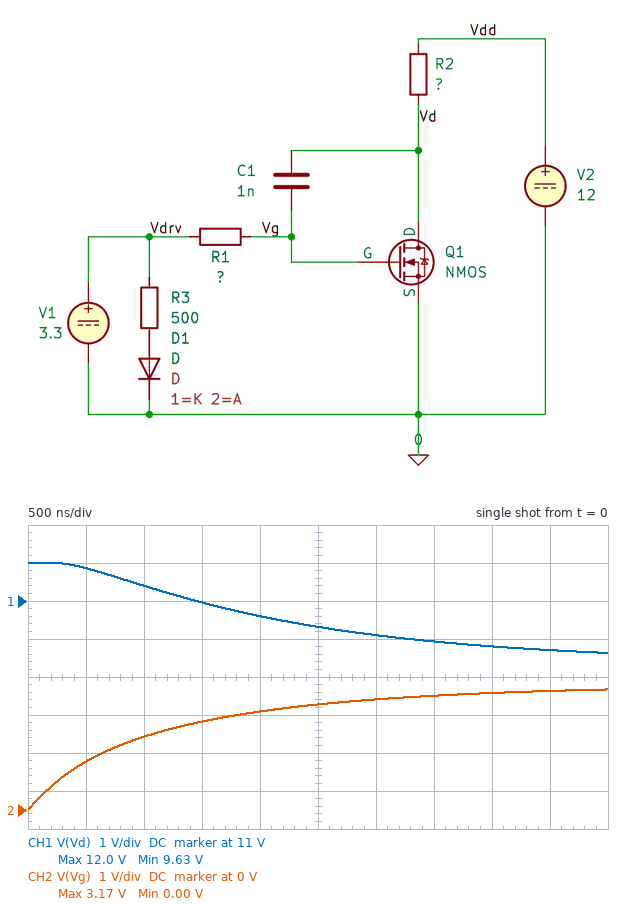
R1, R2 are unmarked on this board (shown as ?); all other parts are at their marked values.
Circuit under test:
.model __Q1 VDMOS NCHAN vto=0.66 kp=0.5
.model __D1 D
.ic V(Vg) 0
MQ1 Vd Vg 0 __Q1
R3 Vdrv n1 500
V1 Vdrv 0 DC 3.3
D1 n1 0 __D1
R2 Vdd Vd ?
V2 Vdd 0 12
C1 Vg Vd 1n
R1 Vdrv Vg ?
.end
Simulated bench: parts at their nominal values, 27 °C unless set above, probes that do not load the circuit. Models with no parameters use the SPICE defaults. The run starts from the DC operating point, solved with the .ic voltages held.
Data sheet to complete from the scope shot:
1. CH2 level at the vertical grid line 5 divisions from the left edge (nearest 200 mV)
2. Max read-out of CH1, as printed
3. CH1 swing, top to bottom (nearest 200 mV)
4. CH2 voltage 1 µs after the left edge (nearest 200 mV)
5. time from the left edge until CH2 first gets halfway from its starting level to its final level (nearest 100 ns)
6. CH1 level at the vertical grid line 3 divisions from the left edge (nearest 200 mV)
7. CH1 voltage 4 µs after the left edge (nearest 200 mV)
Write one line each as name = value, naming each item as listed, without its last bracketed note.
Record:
CH2 level at the vertical grid line 5 divisions from the left edge = 2.8 V
Max read-out of CH1, as printed = 12.0 V
CH1 swing, top to bottom = 2.4 V
CH2 voltage 1 µs after the left edge = 2.0 V
time from the left edge until CH2 first gets halfway from its starting level to its final level = 700 ns
CH1 level at the vertical grid line 3 divisions from the left edge = 11.0 V
CH1 voltage 4 µs after the left edge = 9.8 V
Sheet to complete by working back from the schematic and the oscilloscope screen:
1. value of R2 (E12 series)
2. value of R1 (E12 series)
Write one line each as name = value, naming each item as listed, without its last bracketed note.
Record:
value of R2 = 1.5 Ω
value of R1 = 390 Ω
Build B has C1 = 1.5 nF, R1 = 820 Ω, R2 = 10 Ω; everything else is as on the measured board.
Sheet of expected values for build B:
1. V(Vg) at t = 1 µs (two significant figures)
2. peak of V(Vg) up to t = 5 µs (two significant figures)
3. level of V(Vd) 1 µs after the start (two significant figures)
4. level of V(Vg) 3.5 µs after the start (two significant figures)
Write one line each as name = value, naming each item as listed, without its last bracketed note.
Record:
V(Vg) at t = 1 µs = 980 mV
peak of V(Vg) up to t = 5 µs = 1.9 V
level of V(Vd) 1 µs after the start = 12 V
level of V(Vg) 3.5 µs after the start = 1.7 V
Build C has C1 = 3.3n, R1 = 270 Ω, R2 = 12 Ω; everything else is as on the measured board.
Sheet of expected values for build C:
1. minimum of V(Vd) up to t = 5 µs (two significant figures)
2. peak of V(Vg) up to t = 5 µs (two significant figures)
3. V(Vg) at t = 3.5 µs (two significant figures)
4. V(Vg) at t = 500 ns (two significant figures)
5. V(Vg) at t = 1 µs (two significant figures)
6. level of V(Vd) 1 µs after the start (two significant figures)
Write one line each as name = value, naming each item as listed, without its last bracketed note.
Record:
minimum of V(Vd) up to t = 5 µs = 5.7 V
peak of V(Vg) up to t = 5 µs = 2.1 V
V(Vg) at t = 3.5 µs = 1.9 V
V(Vg) at t = 500 ns = 940 mV
V(Vg) at t = 1 µs = 1.2 V
level of V(Vd) 1 µs after the start = 11 V
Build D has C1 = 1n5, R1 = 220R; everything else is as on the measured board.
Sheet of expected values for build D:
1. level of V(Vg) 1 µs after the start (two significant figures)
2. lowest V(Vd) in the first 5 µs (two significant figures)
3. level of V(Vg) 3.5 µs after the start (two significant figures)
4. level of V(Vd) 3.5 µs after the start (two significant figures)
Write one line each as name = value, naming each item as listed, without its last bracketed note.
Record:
level of V(Vg) 1 µs after the start = 2.3 V
lowest V(Vd) in the first 5 µs = 9.5 V
level of V(Vg) 3.5 µs after the start = 3.2 V
level of V(Vd) 3.5 µs after the start = 9.7 V
